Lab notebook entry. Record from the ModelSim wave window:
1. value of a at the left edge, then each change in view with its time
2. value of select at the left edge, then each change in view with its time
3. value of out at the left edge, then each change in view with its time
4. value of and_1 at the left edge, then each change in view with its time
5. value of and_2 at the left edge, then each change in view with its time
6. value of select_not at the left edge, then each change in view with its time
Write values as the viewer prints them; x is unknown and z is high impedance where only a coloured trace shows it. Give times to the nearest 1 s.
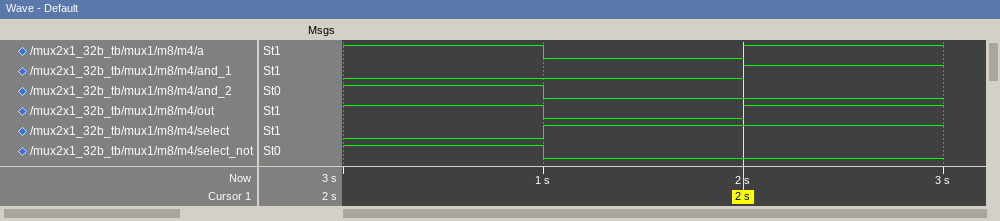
1, 0 at 1 s, 1 at 2 s
0, 1 at 1 s
1, 0 at 1 s, 1 at 2 s
0, 1 at 2 s
1, 0 at 1 s
1, 0 at 1 s
